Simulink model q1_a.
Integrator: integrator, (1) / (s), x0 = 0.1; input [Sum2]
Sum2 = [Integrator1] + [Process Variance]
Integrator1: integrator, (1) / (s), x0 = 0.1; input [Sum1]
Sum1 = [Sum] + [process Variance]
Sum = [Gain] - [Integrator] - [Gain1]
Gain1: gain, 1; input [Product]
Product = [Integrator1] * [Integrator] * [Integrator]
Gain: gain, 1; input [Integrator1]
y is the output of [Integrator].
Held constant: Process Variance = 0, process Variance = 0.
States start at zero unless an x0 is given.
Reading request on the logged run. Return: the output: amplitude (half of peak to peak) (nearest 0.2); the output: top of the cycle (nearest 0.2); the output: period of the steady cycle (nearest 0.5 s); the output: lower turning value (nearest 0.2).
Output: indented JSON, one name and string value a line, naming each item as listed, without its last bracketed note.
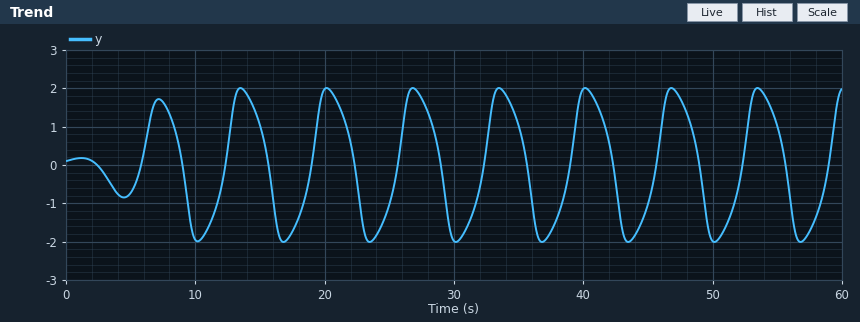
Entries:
{
  "the output: amplitude (half of peak to peak)": "2.0",
  "the output: top of the cycle": "2.0",
  "the output: period of the steady cycle": "6.5 s",
  "the output: lower turning value": "-2.0"
}
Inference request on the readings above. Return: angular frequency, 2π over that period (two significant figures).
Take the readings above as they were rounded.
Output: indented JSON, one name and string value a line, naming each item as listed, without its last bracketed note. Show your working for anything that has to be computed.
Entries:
{
  "angular frequency, 2π over that period": "2π / 6.5 = 0.97 rad/s"
}
